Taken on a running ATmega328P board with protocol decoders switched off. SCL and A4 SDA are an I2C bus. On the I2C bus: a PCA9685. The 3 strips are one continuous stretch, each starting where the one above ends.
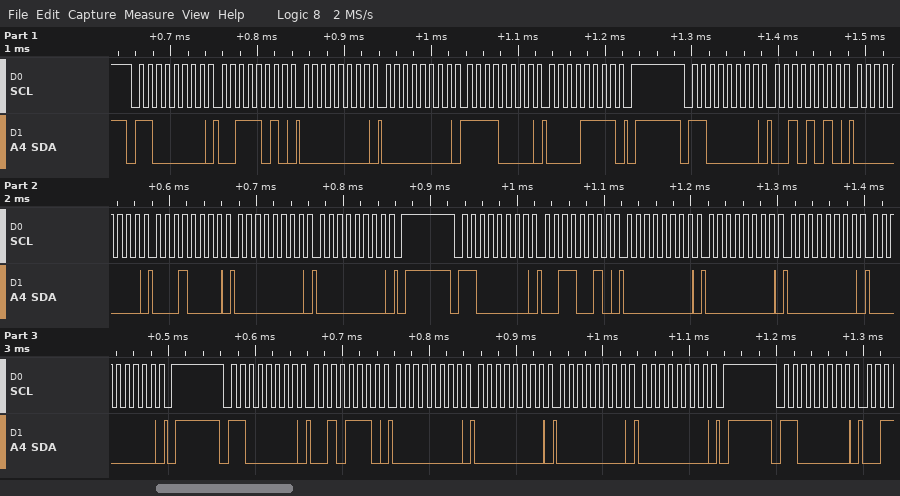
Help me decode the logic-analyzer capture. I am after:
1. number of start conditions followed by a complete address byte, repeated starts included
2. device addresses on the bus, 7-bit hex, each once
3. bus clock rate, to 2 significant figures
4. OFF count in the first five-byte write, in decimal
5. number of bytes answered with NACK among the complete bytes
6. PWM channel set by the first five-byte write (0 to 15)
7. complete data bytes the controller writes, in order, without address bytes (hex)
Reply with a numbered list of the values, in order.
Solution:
1. 5
2. 0x60
3. 100 kHz
4. 4080
5. 0
6. 13
7. 3A 00 00 F0 0F 2A 00 10 00 00 32 00 00 00 00 2E 00 00 00 00
